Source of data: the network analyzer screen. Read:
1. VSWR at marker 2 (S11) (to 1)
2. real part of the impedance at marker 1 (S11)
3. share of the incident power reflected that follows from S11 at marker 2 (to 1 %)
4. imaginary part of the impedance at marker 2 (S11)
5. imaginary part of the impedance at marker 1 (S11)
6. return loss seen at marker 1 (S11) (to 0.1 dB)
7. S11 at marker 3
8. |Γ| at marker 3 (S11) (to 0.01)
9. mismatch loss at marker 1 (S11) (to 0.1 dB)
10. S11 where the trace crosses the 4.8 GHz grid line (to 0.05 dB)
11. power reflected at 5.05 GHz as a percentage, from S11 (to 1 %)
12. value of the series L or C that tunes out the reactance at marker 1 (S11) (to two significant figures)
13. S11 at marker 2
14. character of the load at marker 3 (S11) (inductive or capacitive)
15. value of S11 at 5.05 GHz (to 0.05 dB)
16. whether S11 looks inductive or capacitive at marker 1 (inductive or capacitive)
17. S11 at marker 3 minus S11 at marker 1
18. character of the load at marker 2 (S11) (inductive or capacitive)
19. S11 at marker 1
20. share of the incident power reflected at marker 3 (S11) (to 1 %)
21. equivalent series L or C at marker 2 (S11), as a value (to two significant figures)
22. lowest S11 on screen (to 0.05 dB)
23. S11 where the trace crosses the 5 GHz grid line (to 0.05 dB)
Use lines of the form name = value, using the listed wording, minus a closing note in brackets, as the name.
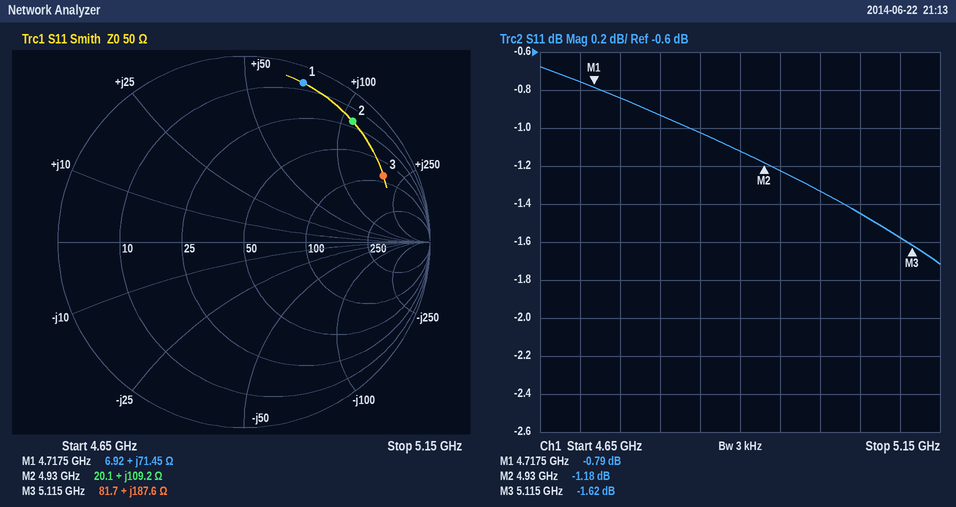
VSWR at marker 2 (S11) = 15
real part of the impedance at marker 1 = 6.92 Ω
share of the incident power reflected that follows from S11 at marker 2 = 76 %
imaginary part of the impedance at marker 2 = +109.2 Ω
imaginary part of the impedance at marker 1 = +71.45 Ω
return loss seen at marker 1 (S11) = 0.8 dB
S11 at marker 3 = -1.62 dB
|Γ| at marker 3 (S11) = 0.83
mismatch loss at marker 1 (S11) = 7.8 dB
S11 where the trace crosses the 4.8 GHz grid line = -0.95 dB
power reflected at 5.05 GHz as a percentage, from S11 = 72 %
value of the series L or C that tunes out the reactance at marker 1 (S11) = 470 fF
S11 at marker 2 = -1.18 dB
character of the load at marker 3 (S11) = inductive
value of S11 at 5.05 GHz = -1.45 dB
whether S11 looks inductive or capacitive at marker 1 = inductive
S11 at marker 3 minus S11 at marker 1 = -0.83 dB
character of the load at marker 2 (S11) = inductive
S11 at marker 1 = -0.79 dB
share of the incident power reflected at marker 3 (S11) = 69 %
equivalent series L or C at marker 2 (S11), as a value = 3.5 nH
lowest S11 on screen = -1.70 dB
S11 where the trace crosses the 5 GHz grid line = -1.35 dB
